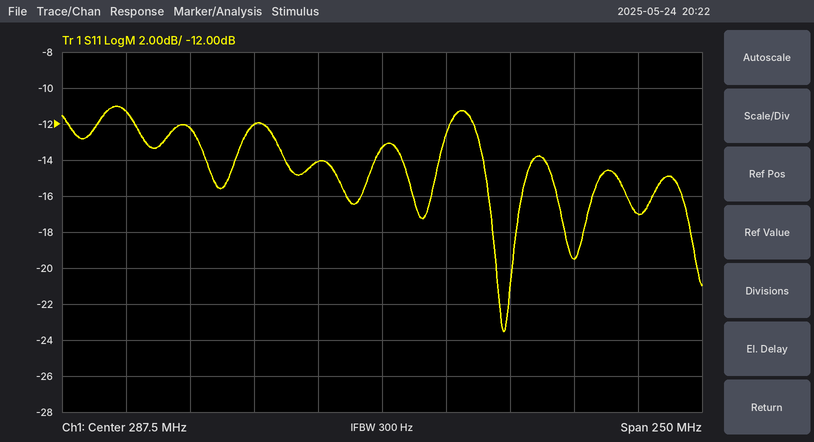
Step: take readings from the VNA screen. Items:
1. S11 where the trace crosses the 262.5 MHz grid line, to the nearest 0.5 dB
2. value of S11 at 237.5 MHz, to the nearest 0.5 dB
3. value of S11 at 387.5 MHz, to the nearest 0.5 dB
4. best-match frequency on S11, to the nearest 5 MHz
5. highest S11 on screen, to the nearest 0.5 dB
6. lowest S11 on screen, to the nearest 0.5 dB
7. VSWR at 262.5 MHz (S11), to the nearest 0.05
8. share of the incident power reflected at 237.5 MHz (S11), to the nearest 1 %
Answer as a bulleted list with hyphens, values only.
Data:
- -14.0 dB
- -12.0 dB
- -17.0 dB
- 335 MHz
- -11.0 dB
- -23.5 dB
- 1.50
- 6 %
